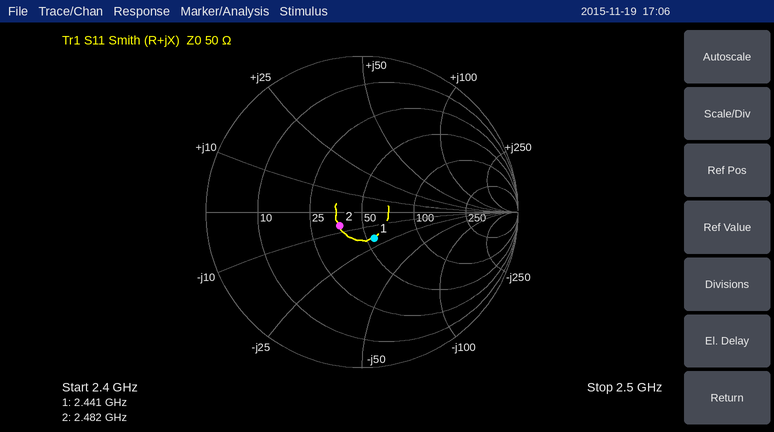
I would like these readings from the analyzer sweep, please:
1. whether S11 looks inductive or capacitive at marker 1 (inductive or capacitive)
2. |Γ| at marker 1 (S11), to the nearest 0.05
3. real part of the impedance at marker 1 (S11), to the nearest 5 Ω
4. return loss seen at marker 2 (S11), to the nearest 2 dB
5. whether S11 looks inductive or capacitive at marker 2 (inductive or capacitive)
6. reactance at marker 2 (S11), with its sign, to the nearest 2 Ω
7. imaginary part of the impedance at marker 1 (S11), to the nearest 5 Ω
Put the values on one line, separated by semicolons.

capacitive; 0.20; 55 Ω; 16 dB; capacitive; -6 Ω; -20 Ω
